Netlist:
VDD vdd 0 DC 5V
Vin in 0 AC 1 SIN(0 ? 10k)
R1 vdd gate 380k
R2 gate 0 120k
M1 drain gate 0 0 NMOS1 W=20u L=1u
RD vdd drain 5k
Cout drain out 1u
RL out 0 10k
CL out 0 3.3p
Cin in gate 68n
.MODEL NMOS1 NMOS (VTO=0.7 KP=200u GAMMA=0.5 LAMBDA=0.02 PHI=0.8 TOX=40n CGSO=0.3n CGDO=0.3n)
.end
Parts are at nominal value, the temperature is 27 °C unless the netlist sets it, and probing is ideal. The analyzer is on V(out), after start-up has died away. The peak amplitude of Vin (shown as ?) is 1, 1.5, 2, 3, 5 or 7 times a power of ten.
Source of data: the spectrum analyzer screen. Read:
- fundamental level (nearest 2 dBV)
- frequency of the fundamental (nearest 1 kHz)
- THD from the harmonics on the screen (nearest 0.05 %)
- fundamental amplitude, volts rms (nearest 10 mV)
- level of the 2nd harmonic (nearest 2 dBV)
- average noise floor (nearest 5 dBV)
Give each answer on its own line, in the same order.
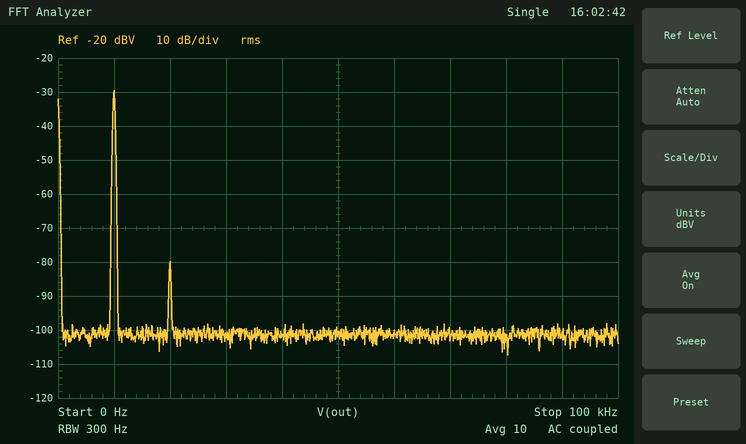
-30 dBV
10 kHz
0.30 %
30 mV
-80 dBV
-100 dBV
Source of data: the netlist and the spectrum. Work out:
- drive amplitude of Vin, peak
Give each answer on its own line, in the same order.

7 mV
